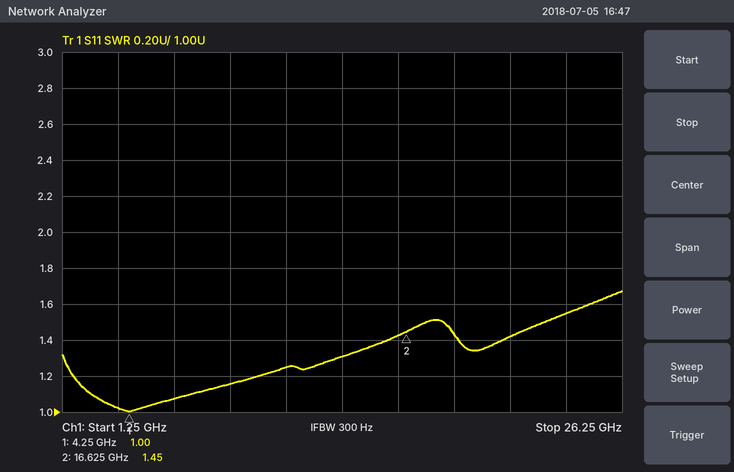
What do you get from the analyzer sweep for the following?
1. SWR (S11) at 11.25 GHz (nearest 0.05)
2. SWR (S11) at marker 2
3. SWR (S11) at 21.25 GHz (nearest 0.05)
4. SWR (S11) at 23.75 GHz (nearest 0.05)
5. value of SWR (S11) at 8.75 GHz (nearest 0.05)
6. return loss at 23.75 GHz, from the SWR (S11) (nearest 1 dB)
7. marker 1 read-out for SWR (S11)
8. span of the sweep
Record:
1.25
1.45
1.40
1.55
1.15
13 dB
1.00
25 GHz
